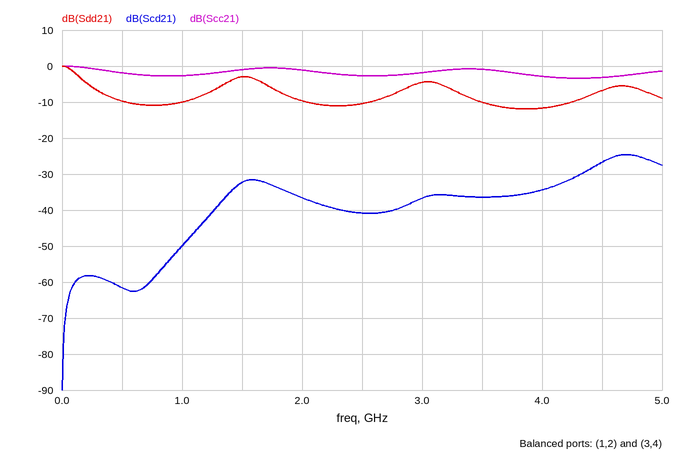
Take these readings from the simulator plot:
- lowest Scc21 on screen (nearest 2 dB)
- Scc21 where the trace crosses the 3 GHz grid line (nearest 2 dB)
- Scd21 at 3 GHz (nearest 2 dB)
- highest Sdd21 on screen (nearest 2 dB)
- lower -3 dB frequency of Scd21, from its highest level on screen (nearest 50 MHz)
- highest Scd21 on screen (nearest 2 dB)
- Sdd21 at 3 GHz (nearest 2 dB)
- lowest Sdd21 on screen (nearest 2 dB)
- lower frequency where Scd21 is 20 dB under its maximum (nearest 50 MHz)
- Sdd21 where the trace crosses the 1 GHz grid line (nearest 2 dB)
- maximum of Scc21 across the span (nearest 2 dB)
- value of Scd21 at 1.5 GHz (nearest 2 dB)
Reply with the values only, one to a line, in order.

-4 dB
-2 dB
-36 dB
0 dB
4.45 GHz
-24 dB
-4 dB
-12 dB
1.15 GHz
-10 dB
0 dB
-32 dB
